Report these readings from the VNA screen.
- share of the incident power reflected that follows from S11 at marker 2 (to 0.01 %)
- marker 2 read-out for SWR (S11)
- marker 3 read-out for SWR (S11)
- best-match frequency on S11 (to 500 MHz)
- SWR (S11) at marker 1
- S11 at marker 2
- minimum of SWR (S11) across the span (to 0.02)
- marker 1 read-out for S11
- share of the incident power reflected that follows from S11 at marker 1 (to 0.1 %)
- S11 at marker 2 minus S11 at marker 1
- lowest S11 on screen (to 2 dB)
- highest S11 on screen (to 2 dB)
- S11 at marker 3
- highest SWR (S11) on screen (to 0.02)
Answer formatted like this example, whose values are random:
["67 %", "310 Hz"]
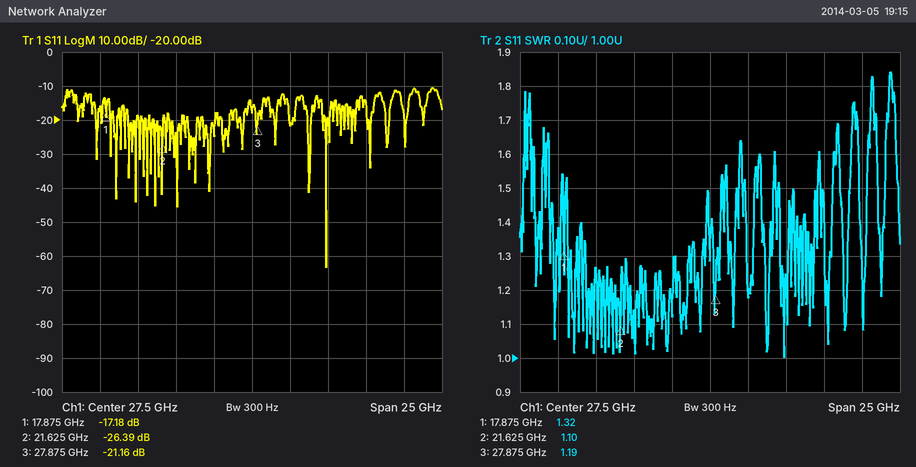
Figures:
["0.23 %", "1.10", "1.19", "32.5 GHz", "1.32", "-26.39 dB", "1.00", "-17.18 dB", "1.9 %", "-9.21 dB", "-64 dB", "-10 dB", "-21.16 dB", "1.84"]
